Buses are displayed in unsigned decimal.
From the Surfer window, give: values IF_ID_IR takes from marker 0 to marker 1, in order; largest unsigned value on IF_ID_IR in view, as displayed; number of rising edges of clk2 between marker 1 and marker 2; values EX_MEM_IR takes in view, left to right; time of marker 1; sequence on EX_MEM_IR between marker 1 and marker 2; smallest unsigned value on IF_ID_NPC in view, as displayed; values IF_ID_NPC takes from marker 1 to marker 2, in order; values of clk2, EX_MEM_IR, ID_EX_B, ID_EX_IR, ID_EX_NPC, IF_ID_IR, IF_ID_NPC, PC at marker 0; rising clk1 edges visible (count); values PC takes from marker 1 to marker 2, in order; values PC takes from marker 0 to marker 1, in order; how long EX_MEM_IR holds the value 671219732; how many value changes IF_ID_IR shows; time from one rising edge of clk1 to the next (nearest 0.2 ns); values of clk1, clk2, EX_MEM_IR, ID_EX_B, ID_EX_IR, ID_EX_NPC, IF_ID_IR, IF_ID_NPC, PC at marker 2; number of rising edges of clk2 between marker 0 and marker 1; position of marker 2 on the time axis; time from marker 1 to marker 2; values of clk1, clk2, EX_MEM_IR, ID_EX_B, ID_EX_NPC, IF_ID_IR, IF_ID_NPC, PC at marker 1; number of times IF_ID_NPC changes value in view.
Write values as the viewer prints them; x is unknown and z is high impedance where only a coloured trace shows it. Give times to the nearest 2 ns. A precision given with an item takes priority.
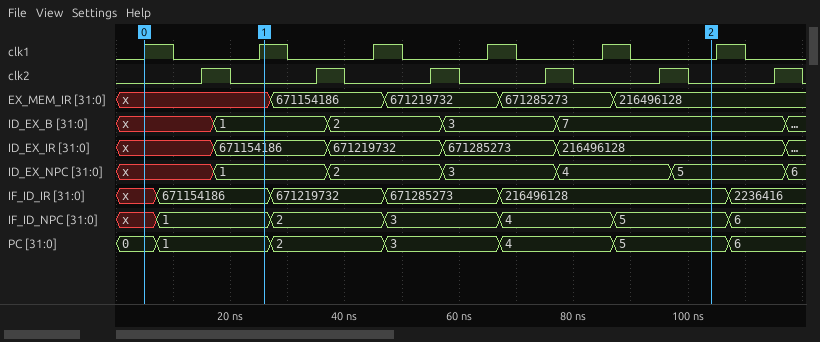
x, 671154186
671285273
4
x, 671154186, 671219732, 671285273, 216496128
26 ns
x, 671154186, 671219732, 671285273, 216496128
1
1, 2, 3, 4, 5
clk2=0, EX_MEM_IR=x, ID_EX_B=x, ID_EX_IR=x, ID_EX_NPC=x, IF_ID_IR=x, IF_ID_NPC=x, PC=0
6
1, 2, 3, 4, 5
0, 1
20 ns
5
20 ns
clk1=0, clk2=0, EX_MEM_IR=216496128, ID_EX_B=7, ID_EX_IR=216496128, ID_EX_NPC=5, IF_ID_IR=216496128, IF_ID_NPC=5, PC=5
1
104 ns
78 ns
clk1=1, clk2=0, EX_MEM_IR=x, ID_EX_B=1, ID_EX_NPC=1, IF_ID_IR=671154186, IF_ID_NPC=1, PC=1
6
